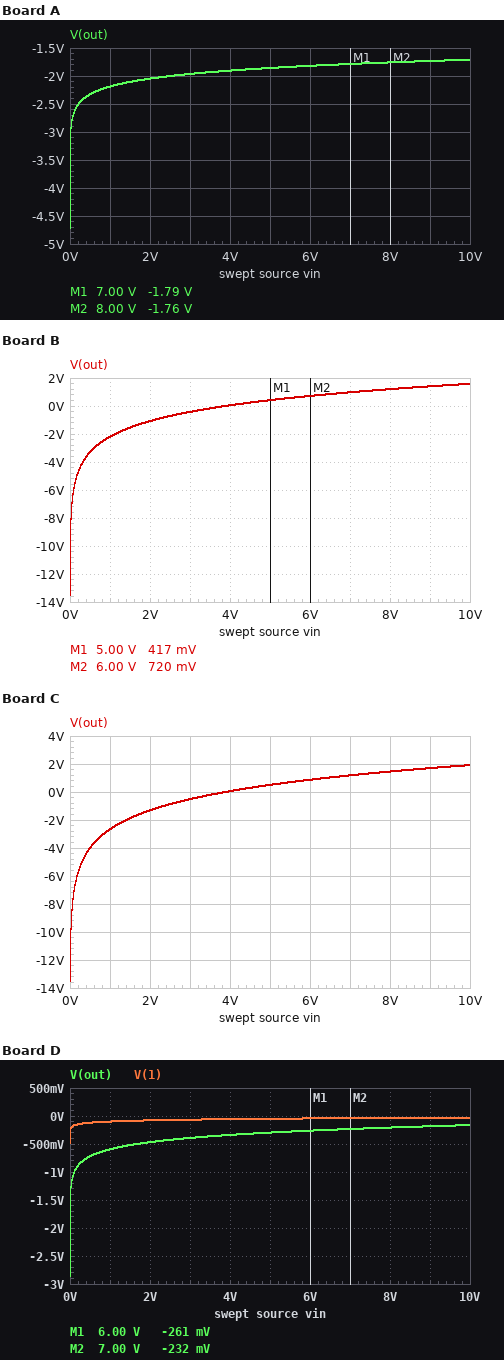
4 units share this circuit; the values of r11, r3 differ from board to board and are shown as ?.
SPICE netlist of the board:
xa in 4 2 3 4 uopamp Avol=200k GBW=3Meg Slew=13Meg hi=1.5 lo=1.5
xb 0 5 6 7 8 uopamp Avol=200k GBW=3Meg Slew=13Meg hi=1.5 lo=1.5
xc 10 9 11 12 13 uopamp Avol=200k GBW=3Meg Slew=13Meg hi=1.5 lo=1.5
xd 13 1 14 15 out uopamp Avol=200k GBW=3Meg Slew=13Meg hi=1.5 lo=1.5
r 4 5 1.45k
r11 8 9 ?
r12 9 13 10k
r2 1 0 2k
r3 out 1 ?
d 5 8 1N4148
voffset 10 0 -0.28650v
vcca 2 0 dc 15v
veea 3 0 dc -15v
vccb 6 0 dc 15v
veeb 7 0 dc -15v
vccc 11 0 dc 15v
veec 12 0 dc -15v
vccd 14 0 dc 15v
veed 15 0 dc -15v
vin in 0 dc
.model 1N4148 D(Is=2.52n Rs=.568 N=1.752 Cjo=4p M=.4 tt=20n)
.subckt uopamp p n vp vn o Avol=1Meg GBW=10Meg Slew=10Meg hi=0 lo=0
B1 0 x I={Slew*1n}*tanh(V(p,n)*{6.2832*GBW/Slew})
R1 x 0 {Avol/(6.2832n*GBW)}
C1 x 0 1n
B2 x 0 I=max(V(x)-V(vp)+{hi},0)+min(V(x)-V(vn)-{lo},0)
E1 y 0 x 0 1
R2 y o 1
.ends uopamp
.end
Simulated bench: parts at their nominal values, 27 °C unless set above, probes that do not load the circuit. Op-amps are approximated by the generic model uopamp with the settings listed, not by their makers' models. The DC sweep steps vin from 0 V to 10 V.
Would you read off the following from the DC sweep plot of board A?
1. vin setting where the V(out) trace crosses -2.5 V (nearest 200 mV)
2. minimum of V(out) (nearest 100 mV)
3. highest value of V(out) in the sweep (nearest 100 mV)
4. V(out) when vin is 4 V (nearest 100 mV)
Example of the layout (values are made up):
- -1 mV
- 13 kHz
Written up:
- 200 mV
- -4.7 V
- -1.7 V
- -1.9 V
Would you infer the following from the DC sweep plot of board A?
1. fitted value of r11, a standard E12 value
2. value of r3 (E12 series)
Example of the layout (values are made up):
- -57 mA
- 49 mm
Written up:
- 27 kΩ
- 22 kΩ
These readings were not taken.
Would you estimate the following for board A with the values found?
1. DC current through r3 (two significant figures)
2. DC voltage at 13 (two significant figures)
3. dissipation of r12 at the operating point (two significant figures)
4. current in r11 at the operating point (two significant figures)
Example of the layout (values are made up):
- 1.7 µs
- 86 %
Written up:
- 200 µA
- -390 mV
- 1.1 µW
- 11 µA
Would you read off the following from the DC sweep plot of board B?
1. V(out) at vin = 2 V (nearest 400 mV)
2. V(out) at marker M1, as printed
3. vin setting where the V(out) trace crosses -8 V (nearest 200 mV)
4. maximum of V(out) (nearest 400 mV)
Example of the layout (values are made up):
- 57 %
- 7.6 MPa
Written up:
- -1.2 V
- 417 mV
- 0 V
- 1.6 V
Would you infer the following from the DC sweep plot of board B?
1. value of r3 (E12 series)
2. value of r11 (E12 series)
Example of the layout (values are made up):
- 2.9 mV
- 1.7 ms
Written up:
- 82 kΩ
- 12 kΩ
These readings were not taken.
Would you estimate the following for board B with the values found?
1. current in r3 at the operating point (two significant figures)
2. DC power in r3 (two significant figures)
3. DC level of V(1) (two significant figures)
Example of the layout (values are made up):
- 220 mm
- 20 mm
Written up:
- 160 µA
- 2.1 mW
- -320 mV
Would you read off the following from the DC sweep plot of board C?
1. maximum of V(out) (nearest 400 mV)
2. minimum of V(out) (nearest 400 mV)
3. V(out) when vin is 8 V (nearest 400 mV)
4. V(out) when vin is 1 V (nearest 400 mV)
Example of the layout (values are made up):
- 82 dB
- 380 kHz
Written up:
- 2.0 V
- -13.6 V
- 1.6 V
- -2.8 V
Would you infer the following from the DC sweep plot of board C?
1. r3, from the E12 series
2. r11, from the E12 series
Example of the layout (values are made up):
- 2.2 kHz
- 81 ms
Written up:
- 100 kΩ
- 12 kΩ
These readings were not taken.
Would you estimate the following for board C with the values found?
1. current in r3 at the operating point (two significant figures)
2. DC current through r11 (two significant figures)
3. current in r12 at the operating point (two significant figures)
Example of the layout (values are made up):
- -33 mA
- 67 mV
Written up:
- 130 µA
- 24 µA
- 24 µA
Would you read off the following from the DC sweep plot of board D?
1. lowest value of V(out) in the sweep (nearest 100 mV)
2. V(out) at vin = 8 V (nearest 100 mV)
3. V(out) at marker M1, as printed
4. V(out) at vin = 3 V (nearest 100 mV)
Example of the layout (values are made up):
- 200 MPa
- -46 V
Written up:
- -2.9 V
- -200 mV
- -261 mV
- -400 mV
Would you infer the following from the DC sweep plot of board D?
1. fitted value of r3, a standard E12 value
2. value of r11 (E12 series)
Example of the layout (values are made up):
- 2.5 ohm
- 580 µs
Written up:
- 10 kΩ
- 15 kΩ
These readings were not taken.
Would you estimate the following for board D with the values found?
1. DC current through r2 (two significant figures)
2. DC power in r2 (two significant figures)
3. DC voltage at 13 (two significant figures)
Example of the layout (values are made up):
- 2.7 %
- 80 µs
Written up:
- 240 µA
- 110 µW
- -480 mV
